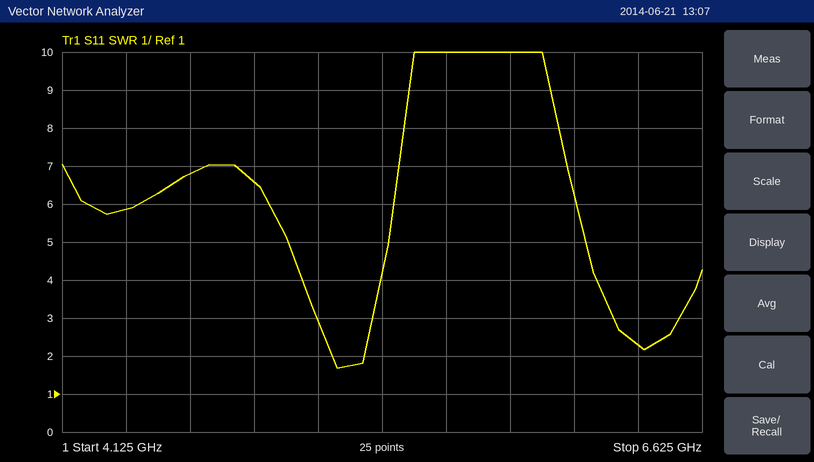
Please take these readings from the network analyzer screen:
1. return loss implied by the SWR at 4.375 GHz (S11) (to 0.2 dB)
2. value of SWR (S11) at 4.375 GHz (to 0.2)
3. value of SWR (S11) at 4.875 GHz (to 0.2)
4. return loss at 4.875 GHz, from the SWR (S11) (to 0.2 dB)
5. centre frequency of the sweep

3.0 dB
5.8
6.6
2.6 dB
5.375 GHz
